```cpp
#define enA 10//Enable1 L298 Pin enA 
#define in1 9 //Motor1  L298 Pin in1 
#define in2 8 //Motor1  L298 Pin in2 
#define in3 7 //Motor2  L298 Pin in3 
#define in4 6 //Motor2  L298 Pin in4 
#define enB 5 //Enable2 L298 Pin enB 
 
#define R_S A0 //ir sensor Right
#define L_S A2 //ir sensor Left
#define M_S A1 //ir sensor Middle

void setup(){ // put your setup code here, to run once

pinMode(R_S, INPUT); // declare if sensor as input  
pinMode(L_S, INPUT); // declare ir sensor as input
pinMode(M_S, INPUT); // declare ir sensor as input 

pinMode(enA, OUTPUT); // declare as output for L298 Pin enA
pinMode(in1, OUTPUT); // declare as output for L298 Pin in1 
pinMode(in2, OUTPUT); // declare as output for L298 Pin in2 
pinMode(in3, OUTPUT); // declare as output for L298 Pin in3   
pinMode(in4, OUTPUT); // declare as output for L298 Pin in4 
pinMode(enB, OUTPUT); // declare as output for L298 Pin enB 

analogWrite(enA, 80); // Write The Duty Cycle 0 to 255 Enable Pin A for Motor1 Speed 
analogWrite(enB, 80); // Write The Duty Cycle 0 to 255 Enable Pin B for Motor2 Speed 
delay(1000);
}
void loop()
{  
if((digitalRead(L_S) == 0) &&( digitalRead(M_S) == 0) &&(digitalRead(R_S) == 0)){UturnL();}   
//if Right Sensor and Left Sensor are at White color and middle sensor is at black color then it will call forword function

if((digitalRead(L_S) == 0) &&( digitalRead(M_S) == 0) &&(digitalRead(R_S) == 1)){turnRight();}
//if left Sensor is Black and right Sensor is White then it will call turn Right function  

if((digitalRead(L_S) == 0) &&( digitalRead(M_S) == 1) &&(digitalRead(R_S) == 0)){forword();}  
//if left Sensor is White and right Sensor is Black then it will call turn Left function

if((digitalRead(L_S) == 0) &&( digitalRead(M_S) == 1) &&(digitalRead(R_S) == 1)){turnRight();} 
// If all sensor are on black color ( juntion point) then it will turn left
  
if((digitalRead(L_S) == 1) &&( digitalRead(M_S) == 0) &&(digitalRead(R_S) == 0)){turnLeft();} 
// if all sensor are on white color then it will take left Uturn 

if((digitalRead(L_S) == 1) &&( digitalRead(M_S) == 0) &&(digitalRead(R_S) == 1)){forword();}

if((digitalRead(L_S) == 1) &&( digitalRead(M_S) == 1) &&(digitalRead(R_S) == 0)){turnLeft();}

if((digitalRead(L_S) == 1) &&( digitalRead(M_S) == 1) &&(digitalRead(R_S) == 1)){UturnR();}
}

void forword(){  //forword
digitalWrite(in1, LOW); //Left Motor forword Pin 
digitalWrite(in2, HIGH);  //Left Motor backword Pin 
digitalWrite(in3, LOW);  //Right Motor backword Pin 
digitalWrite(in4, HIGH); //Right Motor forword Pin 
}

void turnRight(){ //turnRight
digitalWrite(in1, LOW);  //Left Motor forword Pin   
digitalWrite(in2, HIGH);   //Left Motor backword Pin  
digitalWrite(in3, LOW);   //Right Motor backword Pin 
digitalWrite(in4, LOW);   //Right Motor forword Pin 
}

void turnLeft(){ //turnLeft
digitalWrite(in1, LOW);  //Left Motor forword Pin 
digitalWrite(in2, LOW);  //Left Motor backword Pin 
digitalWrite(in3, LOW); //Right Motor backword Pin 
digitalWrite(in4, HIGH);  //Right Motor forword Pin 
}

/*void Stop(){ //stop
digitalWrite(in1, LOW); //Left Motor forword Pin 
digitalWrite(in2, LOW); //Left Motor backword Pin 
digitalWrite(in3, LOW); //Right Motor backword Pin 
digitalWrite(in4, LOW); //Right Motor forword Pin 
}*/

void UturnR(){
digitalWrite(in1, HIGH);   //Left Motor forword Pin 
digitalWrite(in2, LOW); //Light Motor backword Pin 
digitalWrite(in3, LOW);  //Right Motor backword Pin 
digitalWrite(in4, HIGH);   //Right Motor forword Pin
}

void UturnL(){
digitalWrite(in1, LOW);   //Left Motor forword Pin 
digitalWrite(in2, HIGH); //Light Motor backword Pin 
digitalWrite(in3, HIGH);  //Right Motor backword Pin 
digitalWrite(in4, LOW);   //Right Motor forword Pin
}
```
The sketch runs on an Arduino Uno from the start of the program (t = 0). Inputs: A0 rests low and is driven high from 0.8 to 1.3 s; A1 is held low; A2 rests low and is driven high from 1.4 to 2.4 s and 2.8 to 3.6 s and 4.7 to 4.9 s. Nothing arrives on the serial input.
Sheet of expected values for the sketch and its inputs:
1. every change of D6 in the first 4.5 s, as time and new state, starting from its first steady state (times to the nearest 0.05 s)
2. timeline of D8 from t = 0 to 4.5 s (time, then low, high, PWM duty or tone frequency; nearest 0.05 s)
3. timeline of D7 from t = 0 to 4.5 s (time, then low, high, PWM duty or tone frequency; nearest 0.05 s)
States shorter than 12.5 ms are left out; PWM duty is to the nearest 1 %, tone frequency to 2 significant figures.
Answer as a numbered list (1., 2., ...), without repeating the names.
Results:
1. 0 s low; 1.4 s high; 2.4 s low; 2.8 s high; 3.6 s low
2. 0 s low; 1 s high; 1.4 s low; 2.4 s high; 2.8 s low; 3.6 s high
3. 0 s low; 1.3 s high; 1.4 s low; 2.4 s high; 2.8 s low; 3.6 s high
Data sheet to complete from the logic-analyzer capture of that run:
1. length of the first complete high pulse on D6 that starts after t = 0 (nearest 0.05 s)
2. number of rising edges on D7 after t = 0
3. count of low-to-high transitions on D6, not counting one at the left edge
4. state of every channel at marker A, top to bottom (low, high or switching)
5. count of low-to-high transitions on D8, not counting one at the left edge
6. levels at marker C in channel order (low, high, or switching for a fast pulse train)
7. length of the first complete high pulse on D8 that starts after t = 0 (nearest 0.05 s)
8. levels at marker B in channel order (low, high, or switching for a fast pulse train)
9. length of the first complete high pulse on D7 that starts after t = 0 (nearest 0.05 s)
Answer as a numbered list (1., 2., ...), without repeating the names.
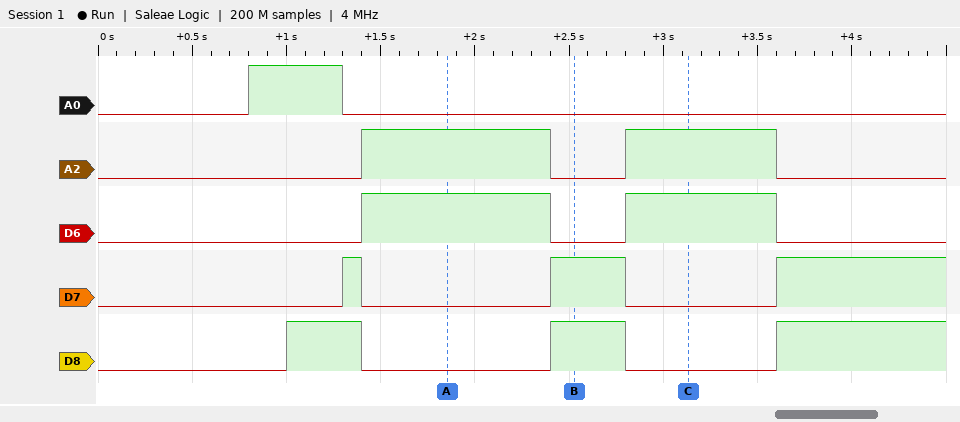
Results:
1. 1.00 s
2. 3
3. 2
4. A0 low, A2 high, D6 high, D7 low, D8 low
5. 3
6. A0 low, A2 high, D6 high, D7 low, D8 low
7. 0.40 s
8. A0 low, A2 low, D6 low, D7 high, D8 high
9. 0.10 s
